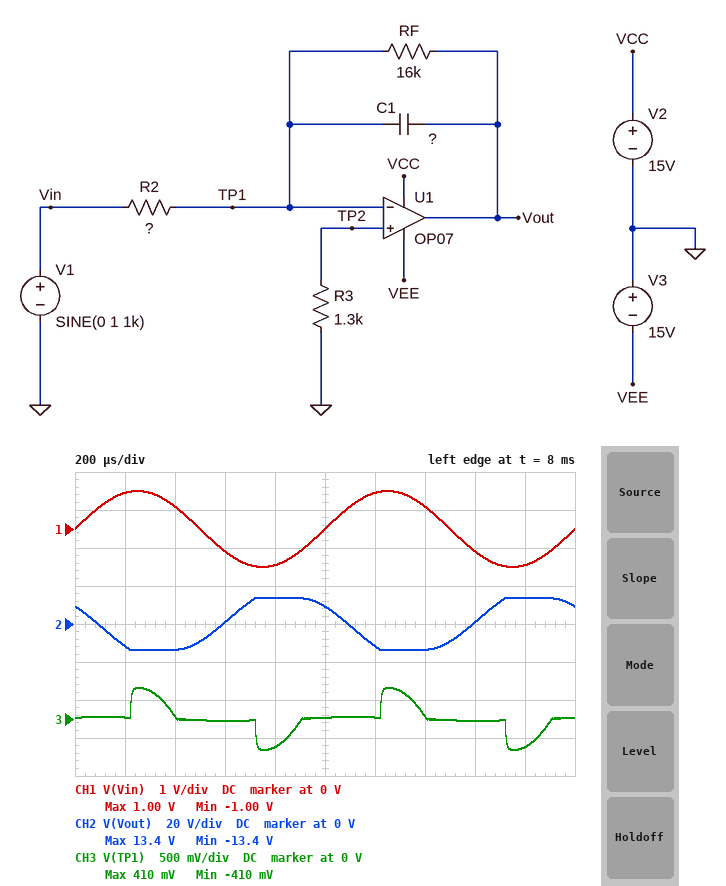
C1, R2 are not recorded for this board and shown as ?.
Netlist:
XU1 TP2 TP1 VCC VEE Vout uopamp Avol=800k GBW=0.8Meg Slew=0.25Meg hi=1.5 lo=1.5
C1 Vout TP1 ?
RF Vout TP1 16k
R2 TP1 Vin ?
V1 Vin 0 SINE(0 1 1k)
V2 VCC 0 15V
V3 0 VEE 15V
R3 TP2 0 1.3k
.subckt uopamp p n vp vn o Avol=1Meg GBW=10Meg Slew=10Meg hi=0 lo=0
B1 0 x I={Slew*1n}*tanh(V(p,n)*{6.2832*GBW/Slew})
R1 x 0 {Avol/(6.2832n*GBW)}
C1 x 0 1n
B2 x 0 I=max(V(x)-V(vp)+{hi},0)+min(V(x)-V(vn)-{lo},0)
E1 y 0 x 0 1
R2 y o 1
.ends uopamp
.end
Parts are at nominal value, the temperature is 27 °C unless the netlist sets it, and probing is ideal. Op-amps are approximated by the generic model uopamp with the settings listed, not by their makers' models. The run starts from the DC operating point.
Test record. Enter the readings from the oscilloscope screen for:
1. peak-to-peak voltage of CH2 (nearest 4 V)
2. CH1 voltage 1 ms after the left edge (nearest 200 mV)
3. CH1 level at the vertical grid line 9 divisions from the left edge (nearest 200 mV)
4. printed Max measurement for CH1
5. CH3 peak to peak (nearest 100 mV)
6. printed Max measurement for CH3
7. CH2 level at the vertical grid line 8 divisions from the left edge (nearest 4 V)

28 V
0 V
-1.0 V
1.00 V
800 mV
410 mV
0 V
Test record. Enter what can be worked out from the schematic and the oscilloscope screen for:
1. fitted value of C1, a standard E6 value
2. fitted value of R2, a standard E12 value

6.8 nF
680 Ω
